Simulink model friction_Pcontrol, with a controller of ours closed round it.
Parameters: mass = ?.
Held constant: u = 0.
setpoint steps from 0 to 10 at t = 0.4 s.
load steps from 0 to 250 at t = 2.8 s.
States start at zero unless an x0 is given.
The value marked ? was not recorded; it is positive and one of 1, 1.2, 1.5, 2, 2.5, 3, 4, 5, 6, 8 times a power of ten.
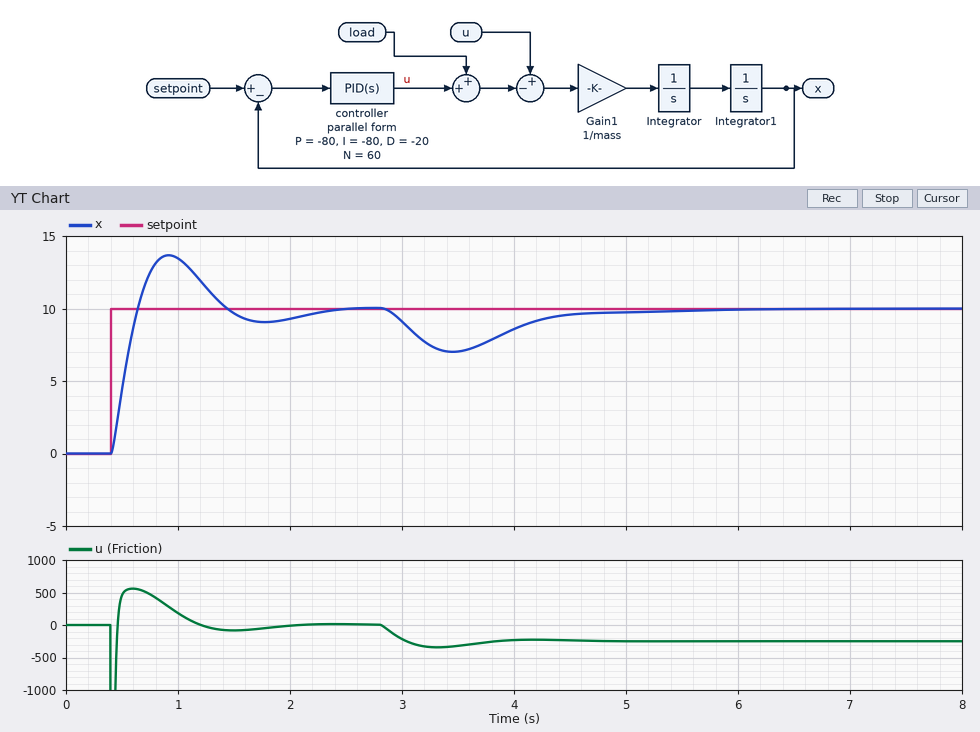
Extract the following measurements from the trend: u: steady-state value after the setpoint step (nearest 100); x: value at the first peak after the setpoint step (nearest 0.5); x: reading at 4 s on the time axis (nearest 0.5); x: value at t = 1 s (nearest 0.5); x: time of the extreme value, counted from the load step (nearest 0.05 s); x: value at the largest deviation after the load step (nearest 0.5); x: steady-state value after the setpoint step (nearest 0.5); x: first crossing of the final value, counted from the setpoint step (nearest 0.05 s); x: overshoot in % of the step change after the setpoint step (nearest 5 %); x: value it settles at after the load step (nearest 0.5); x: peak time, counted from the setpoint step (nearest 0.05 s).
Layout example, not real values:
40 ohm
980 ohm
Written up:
0
13.5
8.5
13.5
0.65 s
7.0
10.0
0.25 s
35 %
10.0
0.50 s
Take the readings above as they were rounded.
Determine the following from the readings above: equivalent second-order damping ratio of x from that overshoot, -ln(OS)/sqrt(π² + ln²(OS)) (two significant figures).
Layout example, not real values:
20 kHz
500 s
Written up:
0.32
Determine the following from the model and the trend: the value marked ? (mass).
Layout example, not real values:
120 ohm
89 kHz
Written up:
4
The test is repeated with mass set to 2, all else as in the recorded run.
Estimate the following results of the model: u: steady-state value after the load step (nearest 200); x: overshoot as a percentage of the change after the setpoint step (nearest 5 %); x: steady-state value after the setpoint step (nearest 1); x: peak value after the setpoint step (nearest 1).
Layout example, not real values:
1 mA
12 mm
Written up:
-200
25 %
10
12
